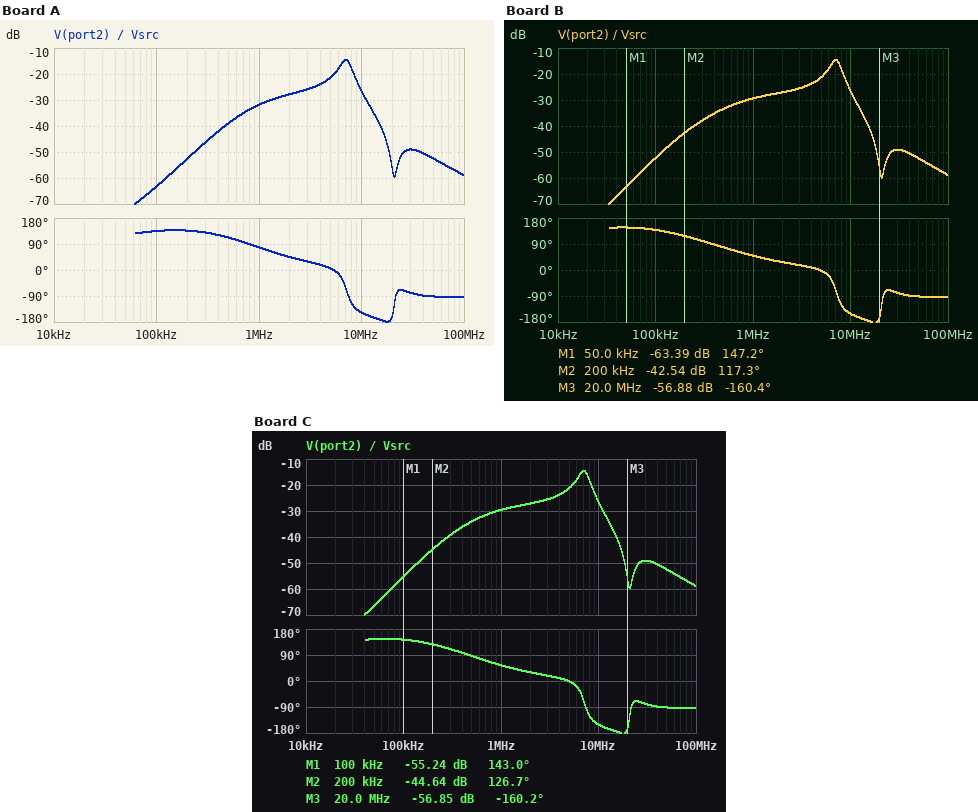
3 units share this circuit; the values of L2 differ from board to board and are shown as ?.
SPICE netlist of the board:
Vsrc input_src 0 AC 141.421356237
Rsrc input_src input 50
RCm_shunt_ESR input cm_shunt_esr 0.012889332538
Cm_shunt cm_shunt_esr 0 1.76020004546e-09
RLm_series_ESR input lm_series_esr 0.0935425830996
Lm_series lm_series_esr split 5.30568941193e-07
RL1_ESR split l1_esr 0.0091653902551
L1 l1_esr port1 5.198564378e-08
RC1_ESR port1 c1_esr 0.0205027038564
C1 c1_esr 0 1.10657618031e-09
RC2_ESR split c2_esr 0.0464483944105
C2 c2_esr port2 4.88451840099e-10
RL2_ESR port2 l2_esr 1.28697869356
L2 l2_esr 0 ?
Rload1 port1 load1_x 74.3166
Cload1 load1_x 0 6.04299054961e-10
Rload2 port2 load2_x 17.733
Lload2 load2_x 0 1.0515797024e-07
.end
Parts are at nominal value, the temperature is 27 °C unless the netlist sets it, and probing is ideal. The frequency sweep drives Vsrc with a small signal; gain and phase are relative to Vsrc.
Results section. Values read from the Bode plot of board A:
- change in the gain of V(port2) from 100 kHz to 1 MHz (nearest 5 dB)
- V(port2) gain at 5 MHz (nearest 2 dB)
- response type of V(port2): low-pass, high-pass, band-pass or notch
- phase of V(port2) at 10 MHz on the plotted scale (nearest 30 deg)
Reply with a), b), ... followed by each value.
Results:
a) 30 dB
b) -22 dB
c) band-pass
d) -150 deg
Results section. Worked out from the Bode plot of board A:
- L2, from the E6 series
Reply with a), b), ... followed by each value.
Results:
a) 3.3 µH
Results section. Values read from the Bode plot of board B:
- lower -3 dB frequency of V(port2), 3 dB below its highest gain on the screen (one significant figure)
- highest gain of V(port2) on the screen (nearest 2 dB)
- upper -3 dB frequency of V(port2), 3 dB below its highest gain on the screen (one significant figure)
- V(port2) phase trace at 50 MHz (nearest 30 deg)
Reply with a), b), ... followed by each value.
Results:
a) 6 MHz
b) -14 dB
c) 8 MHz
d) -90 deg
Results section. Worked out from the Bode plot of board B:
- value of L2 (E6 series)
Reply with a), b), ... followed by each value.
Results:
a) 15 µH
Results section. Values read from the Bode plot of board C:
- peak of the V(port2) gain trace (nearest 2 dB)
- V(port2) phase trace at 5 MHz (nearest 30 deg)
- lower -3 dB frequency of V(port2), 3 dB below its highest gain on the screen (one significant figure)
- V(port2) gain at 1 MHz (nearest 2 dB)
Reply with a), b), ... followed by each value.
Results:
a) -14 dB
b) 0 deg
c) 6 MHz
d) -30 dB
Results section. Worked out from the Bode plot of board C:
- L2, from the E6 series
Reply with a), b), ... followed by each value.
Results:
a) 10 µH
